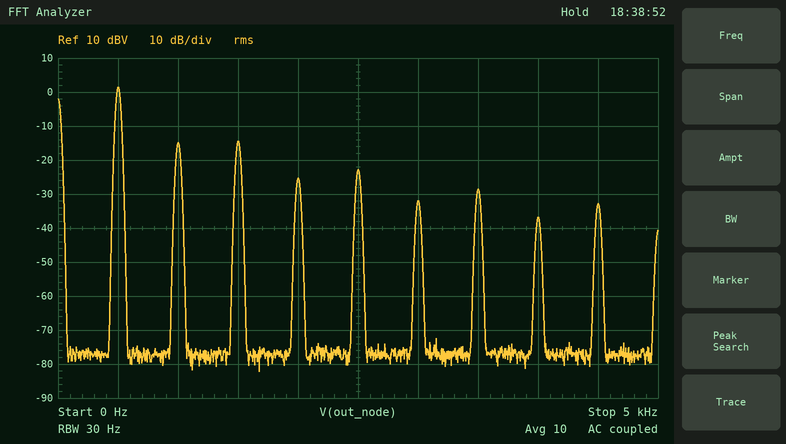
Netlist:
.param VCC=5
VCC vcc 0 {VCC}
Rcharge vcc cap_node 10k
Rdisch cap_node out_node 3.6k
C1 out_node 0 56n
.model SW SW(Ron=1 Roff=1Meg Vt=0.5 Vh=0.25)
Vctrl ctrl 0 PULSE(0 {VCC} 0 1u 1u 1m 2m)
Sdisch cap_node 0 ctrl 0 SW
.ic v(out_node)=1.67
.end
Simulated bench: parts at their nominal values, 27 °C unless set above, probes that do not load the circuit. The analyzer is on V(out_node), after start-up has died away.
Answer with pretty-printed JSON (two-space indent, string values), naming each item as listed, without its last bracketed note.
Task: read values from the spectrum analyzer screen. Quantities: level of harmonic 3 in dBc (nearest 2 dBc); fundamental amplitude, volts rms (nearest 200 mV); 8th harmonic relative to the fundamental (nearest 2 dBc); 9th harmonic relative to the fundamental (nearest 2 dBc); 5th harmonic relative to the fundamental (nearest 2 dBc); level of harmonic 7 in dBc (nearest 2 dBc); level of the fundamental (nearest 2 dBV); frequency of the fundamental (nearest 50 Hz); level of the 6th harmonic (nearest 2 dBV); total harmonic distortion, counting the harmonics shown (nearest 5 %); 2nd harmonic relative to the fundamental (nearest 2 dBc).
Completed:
{
  "level of harmonic 3 in dBc": "-16 dBc",
  "fundamental amplitude, volts rms": "1.2 V",
  "8th harmonic relative to the fundamental": "-38 dBc",
  "9th harmonic relative to the fundamental": "-34 dBc",
  "5th harmonic relative to the fundamental": "-24 dBc",
  "level of harmonic 7 in dBc": "-30 dBc",
  "level of the fundamental": "2 dBV",
  "frequency of the fundamental": "500 Hz",
  "level of the 6th harmonic": "-32 dBV",
  "total harmonic distortion, counting the harmonics shown": "25 %",
  "2nd harmonic relative to the fundamental": "-16 dBc"
}
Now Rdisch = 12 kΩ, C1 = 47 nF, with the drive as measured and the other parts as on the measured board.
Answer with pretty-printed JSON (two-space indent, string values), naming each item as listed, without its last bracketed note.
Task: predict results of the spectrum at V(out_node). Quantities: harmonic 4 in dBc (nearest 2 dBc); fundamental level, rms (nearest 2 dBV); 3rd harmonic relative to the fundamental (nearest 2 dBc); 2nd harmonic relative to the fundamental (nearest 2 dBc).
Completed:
{
  "harmonic 4 in dBc": "-38 dBc",
  "fundamental level, rms": "-2 dBV",
  "3rd harmonic relative to the fundamental": "-18 dBc",
  "2nd harmonic relative to the fundamental": "-26 dBc"
}
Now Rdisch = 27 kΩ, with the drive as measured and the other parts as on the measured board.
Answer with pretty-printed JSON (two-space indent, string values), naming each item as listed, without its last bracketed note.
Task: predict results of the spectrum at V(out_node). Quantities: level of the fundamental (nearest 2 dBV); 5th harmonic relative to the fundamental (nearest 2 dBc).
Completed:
{
  "level of the fundamental": "-8 dBV",
  "5th harmonic relative to the fundamental": "-28 dBc"
}
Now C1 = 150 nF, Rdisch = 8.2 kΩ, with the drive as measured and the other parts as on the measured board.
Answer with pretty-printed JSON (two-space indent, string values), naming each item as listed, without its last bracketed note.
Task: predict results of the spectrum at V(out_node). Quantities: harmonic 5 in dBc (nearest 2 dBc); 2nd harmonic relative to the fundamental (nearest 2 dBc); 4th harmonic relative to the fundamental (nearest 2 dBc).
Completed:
{
  "harmonic 5 in dBc": "-28 dBc",
  "2nd harmonic relative to the fundamental": "-32 dBc",
  "4th harmonic relative to the fundamental": "-44 dBc"
}
